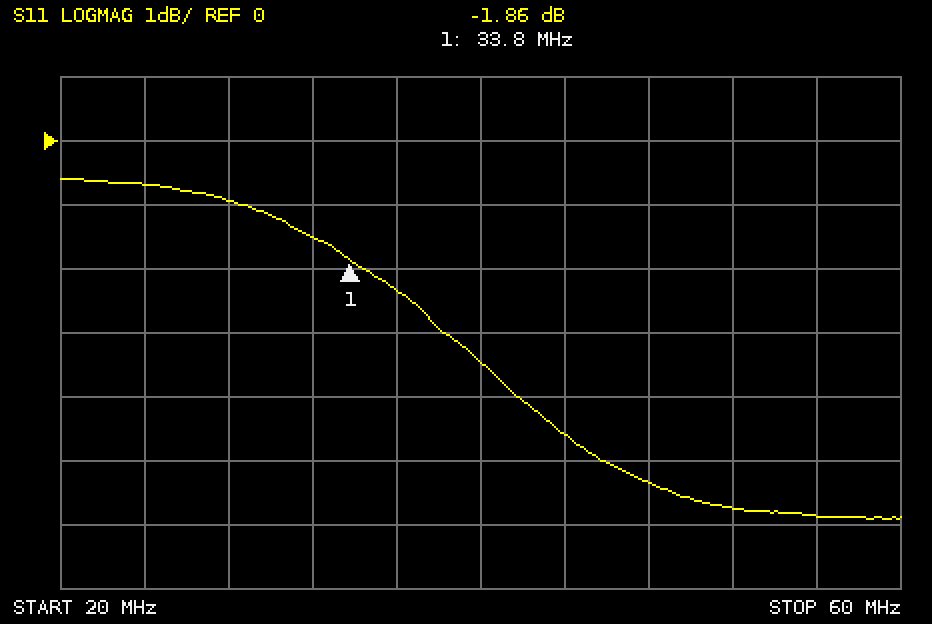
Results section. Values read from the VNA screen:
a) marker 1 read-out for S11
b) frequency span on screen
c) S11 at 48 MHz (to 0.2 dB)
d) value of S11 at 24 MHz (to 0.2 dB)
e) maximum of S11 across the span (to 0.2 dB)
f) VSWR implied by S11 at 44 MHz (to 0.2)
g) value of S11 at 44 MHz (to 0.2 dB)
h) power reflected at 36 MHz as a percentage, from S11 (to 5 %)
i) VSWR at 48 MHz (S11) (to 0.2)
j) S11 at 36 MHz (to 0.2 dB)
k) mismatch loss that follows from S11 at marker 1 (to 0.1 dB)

-1.86 dB
40 MHz
-5.4 dB
-0.6 dB
-0.6 dB
3.8
-4.6 dB
60 %
3.4
-2.4 dB
4.6 dB
